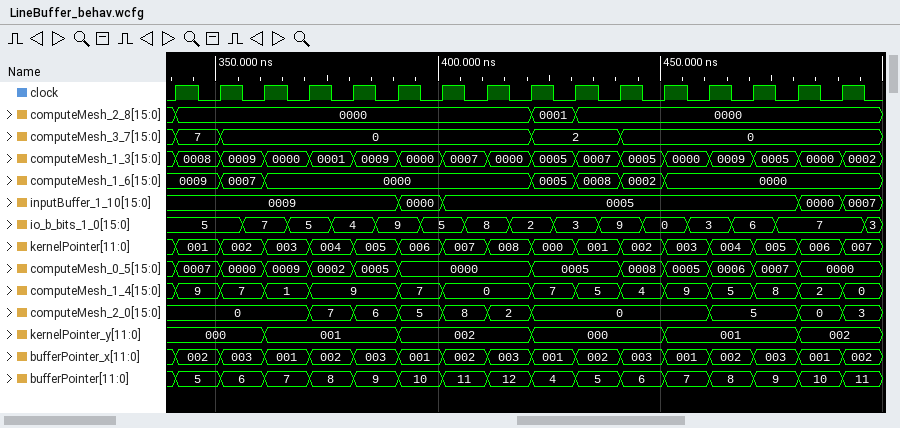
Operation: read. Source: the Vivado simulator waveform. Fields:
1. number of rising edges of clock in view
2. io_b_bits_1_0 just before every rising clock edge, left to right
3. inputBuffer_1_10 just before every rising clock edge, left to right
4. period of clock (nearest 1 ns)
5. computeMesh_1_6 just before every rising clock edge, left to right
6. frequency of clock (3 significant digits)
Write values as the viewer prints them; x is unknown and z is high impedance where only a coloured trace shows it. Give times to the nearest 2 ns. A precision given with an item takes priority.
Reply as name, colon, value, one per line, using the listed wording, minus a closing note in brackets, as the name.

number of rising edges of clock in view: 16
io_b_bits_1_0 just before every rising clock edge, left to right: 5, 5, 7, 5, 4, 9, 5, 8, 2, 3, 9, 0, 3, 6, 7, 7
inputBuffer_1_10 just before every rising clock edge, left to right: 0009, 0009, 0009, 0009, 0009, 0009, 0000, 0005, 0005, 0005, 0005, 0005, 0005, 0005, 0005, 0000
period of clock: 10 ns
computeMesh_1_6 just before every rising clock edge, left to right: 0009, 0009, 0007, 0000, 0000, 0000, 0000, 0000, 0000, 0005, 0008, 0002, 0000, 0000, 0000, 0000
frequency of clock: 100 MHz
